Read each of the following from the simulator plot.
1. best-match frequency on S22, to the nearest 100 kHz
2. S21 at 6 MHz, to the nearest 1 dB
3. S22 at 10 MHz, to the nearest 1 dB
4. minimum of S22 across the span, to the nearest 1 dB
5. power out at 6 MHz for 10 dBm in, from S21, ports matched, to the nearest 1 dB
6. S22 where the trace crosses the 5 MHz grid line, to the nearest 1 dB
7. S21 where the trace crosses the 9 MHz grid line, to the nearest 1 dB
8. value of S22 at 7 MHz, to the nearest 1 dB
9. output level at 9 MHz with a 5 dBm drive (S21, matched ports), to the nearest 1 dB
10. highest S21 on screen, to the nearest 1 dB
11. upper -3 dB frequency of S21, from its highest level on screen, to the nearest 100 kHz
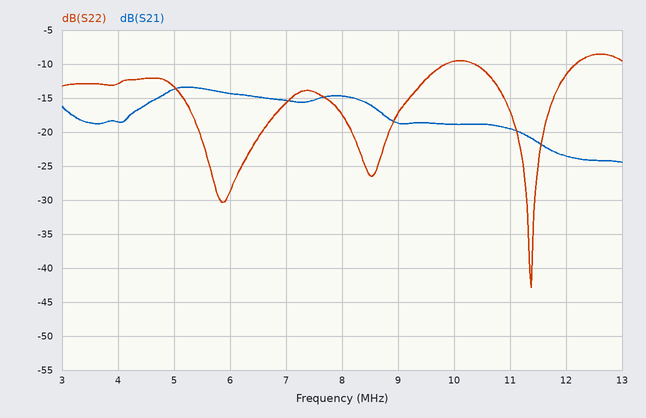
11.4 MHz
-14 dB
-10 dB
-43 dB
-4 dBm
-13 dB
-19 dB
-16 dB
-14 dBm
-13 dB
8.6 MHz
